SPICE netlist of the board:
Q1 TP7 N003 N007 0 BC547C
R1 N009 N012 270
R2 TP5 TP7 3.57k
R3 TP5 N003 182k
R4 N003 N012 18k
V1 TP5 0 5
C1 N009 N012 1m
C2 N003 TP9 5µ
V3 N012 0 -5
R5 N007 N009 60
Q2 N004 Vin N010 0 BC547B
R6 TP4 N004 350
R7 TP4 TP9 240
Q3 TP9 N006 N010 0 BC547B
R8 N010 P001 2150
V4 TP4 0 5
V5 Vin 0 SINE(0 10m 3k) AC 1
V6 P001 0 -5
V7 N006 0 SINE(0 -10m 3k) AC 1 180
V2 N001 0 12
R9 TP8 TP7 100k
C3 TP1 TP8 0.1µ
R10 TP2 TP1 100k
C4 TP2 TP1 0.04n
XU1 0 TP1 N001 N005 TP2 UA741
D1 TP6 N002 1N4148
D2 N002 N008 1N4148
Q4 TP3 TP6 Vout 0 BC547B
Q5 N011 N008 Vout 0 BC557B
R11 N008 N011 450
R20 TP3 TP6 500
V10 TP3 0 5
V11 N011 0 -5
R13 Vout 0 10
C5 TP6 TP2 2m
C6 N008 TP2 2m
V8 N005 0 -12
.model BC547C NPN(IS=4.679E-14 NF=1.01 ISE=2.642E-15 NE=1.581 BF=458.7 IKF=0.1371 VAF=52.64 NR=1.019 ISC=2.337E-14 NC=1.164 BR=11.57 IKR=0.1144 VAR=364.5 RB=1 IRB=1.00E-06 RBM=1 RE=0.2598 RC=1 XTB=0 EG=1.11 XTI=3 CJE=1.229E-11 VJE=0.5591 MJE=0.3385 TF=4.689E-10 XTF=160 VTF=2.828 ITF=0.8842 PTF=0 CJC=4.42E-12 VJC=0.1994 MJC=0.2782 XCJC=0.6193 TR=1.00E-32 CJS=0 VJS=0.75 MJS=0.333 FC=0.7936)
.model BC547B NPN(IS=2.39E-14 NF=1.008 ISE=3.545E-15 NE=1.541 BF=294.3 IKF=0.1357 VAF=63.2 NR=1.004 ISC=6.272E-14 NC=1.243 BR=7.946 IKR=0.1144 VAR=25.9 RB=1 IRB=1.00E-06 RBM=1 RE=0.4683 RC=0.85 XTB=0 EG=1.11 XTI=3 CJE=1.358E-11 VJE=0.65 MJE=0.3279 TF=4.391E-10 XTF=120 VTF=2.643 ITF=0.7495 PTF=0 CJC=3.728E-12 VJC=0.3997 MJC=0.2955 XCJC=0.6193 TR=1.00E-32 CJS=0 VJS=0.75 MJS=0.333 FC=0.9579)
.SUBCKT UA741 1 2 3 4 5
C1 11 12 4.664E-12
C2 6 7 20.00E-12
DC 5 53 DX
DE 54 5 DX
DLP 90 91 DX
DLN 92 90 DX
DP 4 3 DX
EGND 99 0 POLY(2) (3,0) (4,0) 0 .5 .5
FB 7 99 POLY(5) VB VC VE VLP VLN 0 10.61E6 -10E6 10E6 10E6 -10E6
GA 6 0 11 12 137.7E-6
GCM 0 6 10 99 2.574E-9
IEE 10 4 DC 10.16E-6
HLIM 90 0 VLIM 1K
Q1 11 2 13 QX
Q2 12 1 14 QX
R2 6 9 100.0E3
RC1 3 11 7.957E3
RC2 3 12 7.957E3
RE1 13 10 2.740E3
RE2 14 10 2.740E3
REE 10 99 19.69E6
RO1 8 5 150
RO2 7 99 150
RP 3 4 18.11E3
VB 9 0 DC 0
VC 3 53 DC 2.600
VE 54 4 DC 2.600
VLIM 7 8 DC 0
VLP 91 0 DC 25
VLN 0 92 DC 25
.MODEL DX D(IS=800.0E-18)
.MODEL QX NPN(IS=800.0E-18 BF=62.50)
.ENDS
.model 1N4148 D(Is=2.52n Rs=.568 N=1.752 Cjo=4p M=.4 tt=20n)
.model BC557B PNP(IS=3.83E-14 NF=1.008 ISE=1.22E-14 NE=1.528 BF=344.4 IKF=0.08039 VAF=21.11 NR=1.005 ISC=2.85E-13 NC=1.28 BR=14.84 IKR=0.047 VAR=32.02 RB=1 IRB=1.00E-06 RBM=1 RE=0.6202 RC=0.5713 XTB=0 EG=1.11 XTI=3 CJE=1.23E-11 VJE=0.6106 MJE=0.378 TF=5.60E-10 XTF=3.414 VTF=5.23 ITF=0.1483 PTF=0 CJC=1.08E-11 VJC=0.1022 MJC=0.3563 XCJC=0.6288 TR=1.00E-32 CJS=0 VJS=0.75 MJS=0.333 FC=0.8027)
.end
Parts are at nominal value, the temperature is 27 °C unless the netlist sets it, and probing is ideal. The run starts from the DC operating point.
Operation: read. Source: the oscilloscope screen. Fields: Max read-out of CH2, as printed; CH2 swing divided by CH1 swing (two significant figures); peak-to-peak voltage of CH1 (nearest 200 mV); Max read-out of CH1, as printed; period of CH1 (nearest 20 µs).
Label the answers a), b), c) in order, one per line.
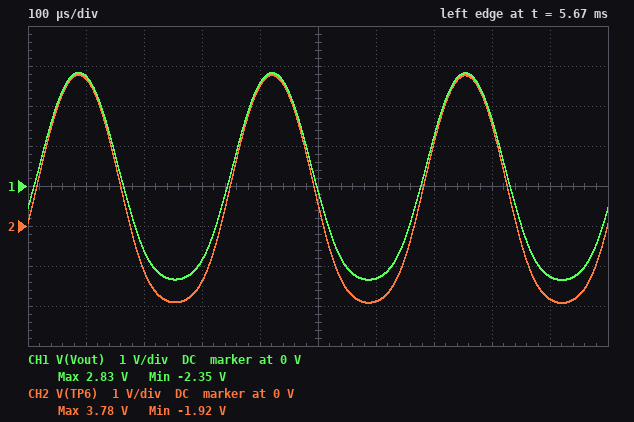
a) 3.78 V
b) 1.1
c) 5.2 V
d) 2.83 V
e) 340 µs
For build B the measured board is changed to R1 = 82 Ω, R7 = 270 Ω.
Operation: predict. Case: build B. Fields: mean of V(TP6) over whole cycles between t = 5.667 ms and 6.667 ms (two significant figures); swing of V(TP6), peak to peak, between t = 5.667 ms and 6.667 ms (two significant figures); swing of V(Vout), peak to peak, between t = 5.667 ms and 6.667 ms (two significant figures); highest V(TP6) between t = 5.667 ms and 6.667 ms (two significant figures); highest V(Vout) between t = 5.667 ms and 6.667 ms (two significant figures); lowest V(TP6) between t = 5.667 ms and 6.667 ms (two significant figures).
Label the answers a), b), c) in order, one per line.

a) 520 mV
b) 7.8 V
c) 7.1 V
d) 4.6 V
e) 3.6 V
f) -3.2 V
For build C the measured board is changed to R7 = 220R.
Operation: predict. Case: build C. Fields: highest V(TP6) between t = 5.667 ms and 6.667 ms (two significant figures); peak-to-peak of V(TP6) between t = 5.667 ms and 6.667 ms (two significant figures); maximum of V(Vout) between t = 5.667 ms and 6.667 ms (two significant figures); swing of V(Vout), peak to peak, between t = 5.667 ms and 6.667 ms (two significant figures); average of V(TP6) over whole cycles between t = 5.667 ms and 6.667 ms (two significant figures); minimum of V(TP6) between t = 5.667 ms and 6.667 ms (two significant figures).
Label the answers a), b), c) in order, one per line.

a) 3.5 V
b) 5.3 V
c) 2.6 V
d) 4.8 V
e) 600 mV
f) -1.8 V
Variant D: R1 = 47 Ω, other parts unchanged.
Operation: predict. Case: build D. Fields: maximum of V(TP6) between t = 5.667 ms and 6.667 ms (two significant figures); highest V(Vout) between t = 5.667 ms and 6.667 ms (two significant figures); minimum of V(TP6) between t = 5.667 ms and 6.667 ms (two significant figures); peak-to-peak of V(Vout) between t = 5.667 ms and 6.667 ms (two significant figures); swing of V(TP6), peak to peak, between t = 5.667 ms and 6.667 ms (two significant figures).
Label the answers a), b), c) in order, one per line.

a) 3.6 V
b) 2.7 V
c) -3.2 V
d) 6.2 V
e) 6.8 V
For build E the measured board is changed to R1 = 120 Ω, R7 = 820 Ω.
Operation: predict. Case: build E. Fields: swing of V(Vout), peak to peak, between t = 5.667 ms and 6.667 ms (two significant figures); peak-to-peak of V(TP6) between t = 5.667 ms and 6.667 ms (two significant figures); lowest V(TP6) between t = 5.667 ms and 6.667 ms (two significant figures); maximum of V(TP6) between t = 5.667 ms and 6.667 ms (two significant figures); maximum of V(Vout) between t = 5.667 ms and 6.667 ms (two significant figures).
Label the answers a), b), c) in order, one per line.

a) 8.2 V
b) 8.9 V
c) -3.8 V
d) 5.1 V
e) 4.1 V
